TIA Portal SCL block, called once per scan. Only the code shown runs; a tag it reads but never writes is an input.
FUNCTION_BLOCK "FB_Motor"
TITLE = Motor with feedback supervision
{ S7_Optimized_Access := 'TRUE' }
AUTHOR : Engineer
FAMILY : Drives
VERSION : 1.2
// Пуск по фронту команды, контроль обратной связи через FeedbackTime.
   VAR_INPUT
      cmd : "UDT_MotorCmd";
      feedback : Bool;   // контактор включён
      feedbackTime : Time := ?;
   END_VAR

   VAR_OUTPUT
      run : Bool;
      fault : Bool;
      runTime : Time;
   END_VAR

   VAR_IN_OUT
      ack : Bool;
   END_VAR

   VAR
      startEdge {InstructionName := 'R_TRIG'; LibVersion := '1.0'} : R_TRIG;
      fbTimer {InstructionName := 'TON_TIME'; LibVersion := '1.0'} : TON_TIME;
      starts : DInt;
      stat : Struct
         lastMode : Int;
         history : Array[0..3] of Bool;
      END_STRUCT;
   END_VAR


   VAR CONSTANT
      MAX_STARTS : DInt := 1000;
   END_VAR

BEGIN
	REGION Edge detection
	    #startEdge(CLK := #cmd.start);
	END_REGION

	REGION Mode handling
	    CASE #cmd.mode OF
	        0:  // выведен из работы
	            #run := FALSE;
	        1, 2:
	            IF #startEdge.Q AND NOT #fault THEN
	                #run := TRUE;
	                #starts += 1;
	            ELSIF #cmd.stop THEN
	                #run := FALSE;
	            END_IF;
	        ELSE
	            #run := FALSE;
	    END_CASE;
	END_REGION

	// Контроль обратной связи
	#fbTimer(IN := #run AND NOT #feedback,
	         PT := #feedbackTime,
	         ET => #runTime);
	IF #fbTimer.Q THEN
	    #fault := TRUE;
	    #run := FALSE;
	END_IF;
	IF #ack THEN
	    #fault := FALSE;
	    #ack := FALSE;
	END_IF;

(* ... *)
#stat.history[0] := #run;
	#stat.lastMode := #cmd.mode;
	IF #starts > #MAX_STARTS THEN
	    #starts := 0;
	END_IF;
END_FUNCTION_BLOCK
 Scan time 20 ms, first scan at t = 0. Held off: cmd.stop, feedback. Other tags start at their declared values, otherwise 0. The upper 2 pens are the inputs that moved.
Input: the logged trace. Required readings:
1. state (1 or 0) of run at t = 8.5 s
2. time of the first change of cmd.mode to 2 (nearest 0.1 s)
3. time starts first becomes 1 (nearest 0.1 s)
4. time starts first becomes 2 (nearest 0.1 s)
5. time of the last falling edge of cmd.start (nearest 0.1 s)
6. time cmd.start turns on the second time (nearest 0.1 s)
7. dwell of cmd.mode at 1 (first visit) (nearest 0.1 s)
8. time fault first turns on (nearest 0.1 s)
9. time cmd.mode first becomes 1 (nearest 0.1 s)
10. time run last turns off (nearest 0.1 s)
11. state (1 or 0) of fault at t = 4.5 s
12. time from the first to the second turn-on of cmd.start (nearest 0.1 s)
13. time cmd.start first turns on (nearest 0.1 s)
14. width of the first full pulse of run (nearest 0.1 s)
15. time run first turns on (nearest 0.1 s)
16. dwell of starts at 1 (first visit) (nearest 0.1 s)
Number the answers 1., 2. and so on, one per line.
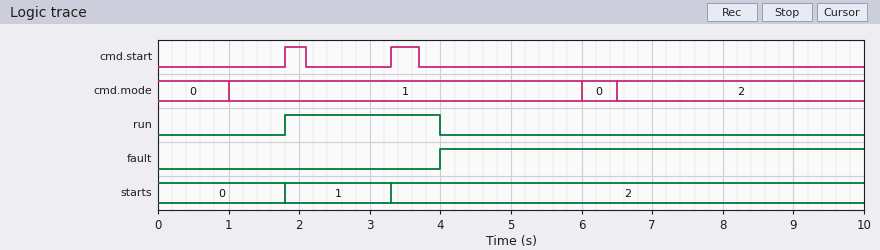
1. 0
2. 6.5 s
3. 1.8 s
4. 3.3 s
5. 3.7 s
6. 3.3 s
7. 5.0 s
8. 4.0 s
9. 1.0 s
10. 4.0 s
11. 1
12. 1.5 s
13. 1.8 s
14. 2.2 s
15. 1.8 s
16. 1.5 s
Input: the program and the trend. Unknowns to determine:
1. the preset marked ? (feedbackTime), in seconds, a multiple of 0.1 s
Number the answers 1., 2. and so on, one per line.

1. 2.2 s
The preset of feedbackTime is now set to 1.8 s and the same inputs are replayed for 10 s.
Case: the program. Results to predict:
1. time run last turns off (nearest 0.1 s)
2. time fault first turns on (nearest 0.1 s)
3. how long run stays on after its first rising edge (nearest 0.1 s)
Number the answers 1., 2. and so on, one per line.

1. 3.6 s
2. 3.6 s
3. 1.8 s
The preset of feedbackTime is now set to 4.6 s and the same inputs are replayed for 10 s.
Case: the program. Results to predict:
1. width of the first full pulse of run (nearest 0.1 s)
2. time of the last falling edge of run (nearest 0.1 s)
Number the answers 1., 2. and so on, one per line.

1. 4.2 s
2. 6.0 s
